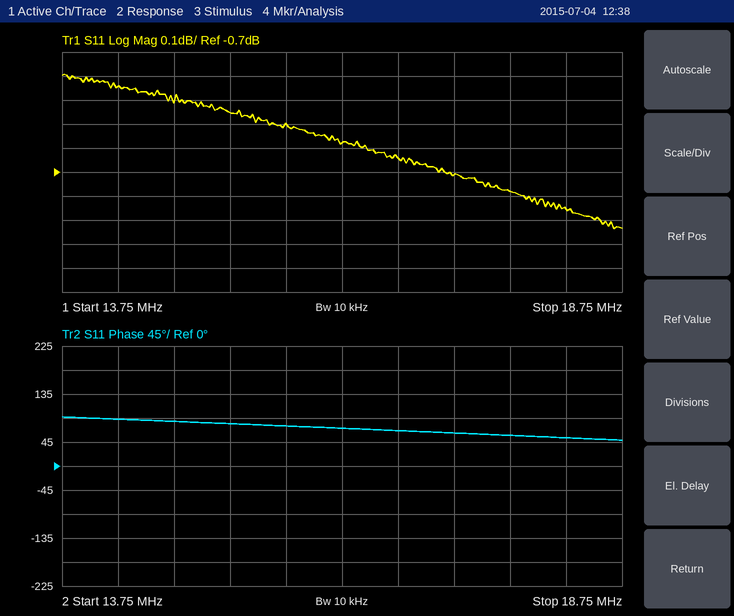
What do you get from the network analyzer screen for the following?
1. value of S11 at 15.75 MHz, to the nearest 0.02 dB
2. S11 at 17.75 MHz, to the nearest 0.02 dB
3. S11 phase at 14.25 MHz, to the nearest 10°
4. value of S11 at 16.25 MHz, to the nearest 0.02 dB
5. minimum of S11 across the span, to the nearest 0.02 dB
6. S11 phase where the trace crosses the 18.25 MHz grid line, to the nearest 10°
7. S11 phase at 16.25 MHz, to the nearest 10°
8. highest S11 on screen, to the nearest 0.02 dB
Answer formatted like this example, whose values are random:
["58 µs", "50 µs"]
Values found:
["-0.50 dB", "-0.78 dB", "90°", "-0.58 dB", "-0.94 dB", "50°", "70°", "-0.30 dB"]
